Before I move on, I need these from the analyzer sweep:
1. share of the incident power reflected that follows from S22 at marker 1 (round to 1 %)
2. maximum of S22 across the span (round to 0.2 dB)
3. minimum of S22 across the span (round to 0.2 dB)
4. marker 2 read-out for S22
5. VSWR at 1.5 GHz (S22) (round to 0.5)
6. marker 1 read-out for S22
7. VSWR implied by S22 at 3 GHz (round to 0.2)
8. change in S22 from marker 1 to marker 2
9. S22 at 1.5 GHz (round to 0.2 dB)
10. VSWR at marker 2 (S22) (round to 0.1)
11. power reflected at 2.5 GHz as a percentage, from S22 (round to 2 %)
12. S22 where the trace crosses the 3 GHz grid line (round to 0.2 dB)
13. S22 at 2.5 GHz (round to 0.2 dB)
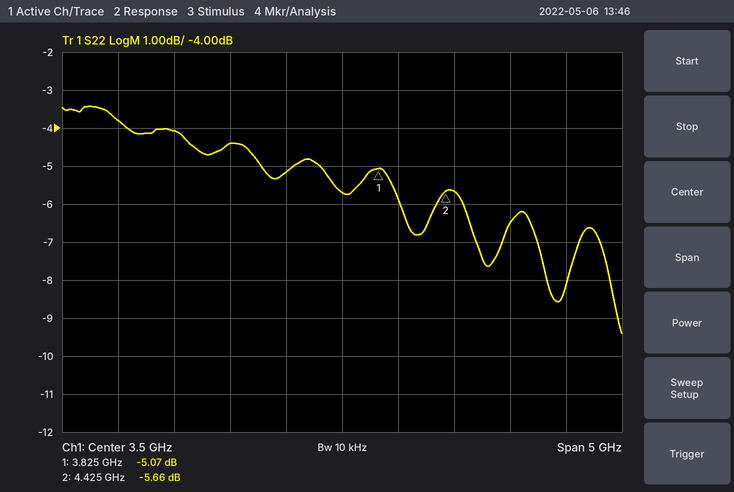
31 %
-3.4 dB
-9.4 dB
-5.66 dB
4.5
-5.07 dB
3.4
-0.59 dB
-3.8 dB
3.2
36 %
-5.2 dB
-4.4 dB
